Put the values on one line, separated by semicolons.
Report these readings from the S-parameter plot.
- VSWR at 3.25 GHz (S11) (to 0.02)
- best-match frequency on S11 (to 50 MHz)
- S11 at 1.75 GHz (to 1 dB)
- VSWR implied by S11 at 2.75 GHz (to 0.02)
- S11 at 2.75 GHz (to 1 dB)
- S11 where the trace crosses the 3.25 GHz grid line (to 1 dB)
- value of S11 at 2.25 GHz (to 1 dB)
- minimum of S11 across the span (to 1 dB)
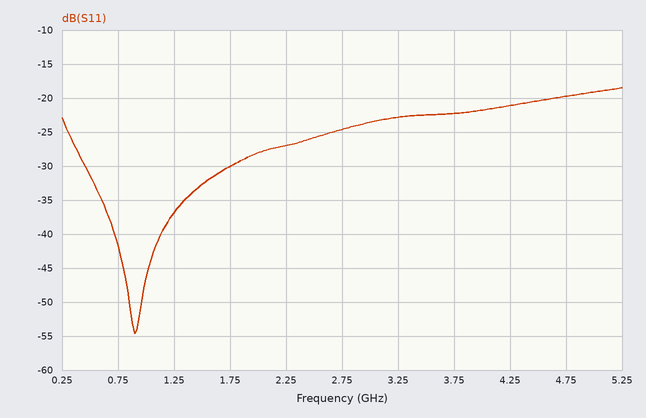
1.16; 900 MHz; -30 dB; 1.12; -25 dB; -23 dB; -27 dB; -55 dB
